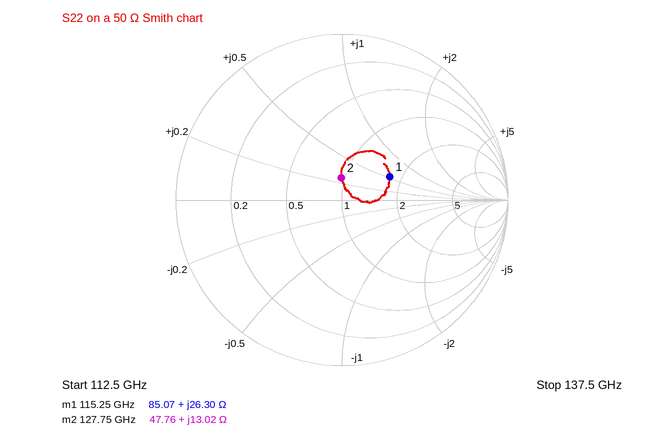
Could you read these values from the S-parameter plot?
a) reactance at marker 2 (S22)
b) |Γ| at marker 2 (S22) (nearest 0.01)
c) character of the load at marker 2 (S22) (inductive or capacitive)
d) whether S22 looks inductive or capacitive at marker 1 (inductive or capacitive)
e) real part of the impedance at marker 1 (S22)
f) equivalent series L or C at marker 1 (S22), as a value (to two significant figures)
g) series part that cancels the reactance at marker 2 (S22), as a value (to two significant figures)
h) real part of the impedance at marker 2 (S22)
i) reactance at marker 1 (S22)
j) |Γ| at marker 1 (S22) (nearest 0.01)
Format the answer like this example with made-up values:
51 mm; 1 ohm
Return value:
+13.02 Ω; 0.13; inductive; inductive; 85.07 Ω; 36 pH; 96 fF; 47.76 Ω; +26.30 Ω; 0.32
